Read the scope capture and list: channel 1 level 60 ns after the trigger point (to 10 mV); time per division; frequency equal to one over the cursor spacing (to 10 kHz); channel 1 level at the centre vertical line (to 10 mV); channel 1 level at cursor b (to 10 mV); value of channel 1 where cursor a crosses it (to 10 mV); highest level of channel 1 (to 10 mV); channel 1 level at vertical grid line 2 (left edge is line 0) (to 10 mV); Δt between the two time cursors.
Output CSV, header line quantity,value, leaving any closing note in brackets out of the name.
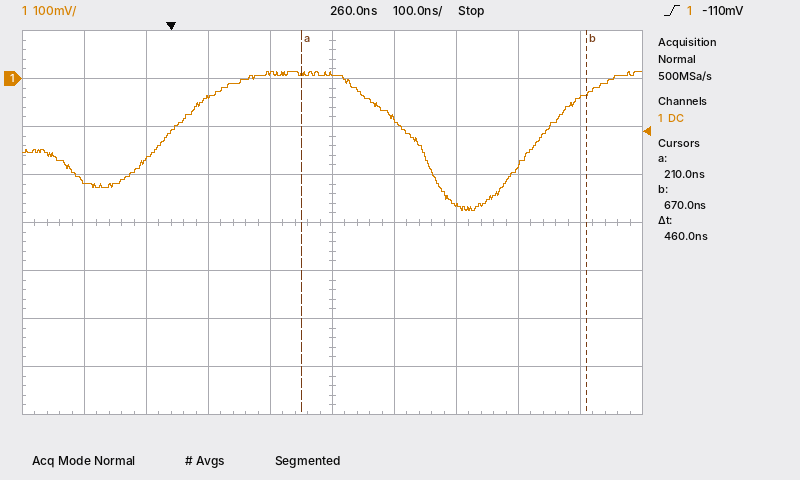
quantity,value
channel 1 level 60 ns after the trigger point,-40 mV
time per division,100 ns
frequency equal to one over the cursor spacing,2.17 MHz
channel 1 level at the centre vertical line,10 mV
channel 1 level at cursor b,-30 mV
value of channel 1 where cursor a crosses it,10 mV
highest level of channel 1,10 mV
channel 1 level at vertical grid line 2 (left edge is line 0),-170 mV
Δt between the two time cursors,460 ns
